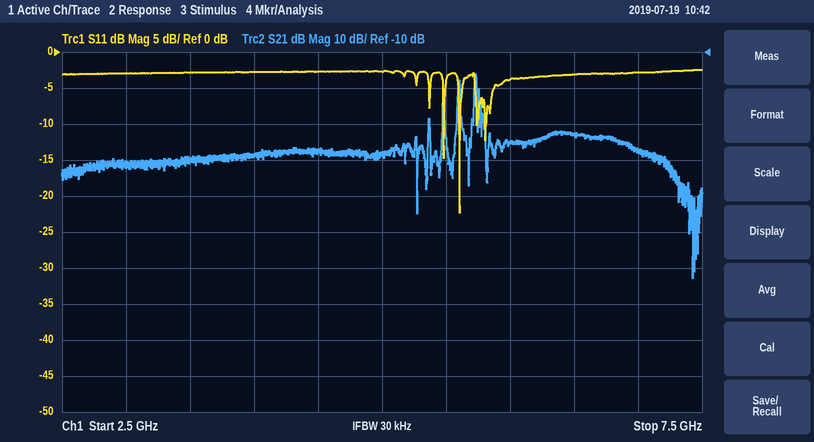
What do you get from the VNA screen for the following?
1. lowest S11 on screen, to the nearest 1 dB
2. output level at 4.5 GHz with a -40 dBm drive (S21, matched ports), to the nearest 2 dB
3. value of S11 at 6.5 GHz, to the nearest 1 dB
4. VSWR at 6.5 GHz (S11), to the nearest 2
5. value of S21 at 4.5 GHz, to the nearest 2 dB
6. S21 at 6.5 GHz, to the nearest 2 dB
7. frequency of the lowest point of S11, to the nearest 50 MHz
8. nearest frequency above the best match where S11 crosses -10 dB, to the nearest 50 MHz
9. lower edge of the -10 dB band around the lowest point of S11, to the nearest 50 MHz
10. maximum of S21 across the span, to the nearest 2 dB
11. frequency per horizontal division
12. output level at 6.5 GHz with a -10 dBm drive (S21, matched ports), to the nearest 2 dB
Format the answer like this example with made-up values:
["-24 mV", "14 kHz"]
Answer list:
["-22 dB", "-78 dBm", "-3 dB", "6", "-38 dB", "-32 dB", "5.60 GHz", "5.60 GHz", "5.60 GHz", "-16 dB", "500 MHz", "-42 dBm"]
